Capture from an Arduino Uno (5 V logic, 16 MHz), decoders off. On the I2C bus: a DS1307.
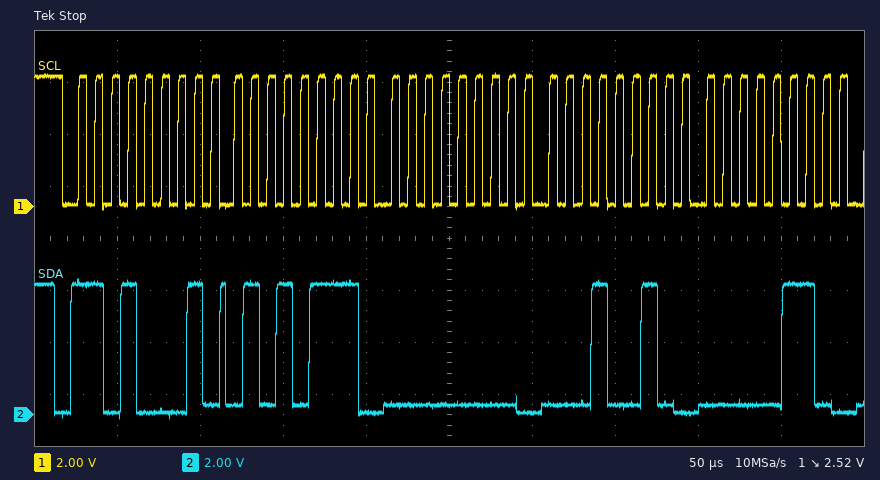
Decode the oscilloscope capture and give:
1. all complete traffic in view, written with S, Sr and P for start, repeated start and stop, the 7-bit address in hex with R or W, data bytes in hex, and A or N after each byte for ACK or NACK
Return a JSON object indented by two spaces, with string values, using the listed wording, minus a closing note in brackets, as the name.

{
  "all complete traffic in view, written with S, Sr and P for start, repeated start and stop, the 7-bit address in hex with R or W, data bytes in hex, and A or N after each byte for ACK or NACK": "S 68R A 57 A 00 A 12 A 06 A"
}
